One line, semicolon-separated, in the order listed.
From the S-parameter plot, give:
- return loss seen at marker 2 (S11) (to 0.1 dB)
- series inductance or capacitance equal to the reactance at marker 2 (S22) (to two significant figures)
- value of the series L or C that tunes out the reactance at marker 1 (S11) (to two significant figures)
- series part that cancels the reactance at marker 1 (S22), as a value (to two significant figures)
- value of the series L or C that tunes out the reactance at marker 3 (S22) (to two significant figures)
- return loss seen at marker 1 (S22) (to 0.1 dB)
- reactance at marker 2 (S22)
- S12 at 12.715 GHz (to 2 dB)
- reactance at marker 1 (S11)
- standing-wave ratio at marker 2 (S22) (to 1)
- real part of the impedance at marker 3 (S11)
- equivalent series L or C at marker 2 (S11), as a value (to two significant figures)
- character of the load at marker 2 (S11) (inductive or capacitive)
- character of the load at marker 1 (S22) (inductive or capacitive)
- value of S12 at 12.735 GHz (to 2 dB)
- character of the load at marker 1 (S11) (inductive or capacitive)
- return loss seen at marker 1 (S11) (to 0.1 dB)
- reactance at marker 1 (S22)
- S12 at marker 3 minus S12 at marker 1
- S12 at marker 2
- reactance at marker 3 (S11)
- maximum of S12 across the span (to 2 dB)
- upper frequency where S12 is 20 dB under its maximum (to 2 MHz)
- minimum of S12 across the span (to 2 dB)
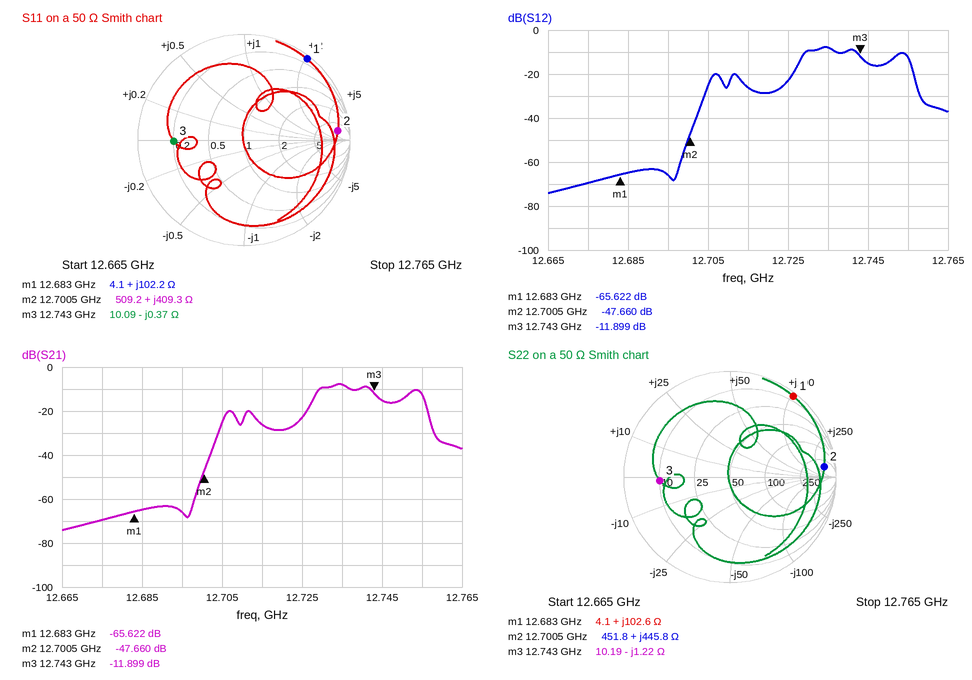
1.0 dB; 5.6 nH; 120 fF; 120 fF; 15 pH; 0.3 dB; +445.8 Ω; -26 dB; +102.2 Ω; 18; 10.09 Ω; 5.1 nH; inductive; inductive; -8 dB; inductive; 0.3 dB; +102.6 Ω; 53.723 dB; -47.660 dB; -0.37 Ω; -8 dB; 12.758 GHz; -74 dB
